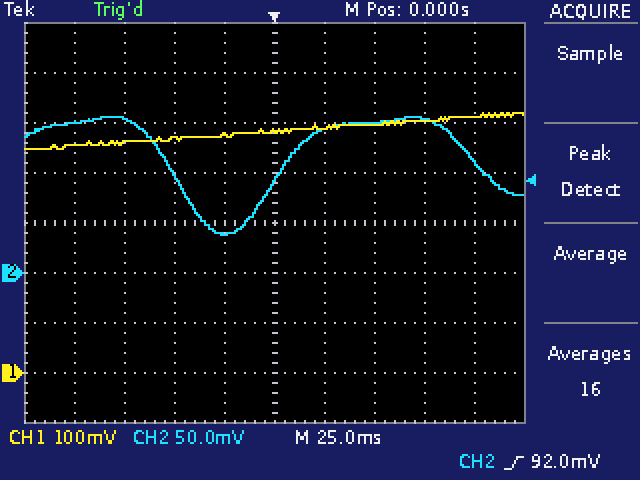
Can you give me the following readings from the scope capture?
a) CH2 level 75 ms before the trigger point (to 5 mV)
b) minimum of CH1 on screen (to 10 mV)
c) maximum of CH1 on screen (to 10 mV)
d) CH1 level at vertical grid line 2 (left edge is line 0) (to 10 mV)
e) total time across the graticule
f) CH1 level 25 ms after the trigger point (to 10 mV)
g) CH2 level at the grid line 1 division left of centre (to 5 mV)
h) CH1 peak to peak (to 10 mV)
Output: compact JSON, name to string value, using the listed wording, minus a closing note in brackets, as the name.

{"CH2 level 75 ms before the trigger point": "155 mV", "minimum of CH1 on screen": "450 mV", "maximum of CH1 on screen": "520 mV", "CH1 level at vertical grid line 2 (left edge is line 0)": "460 mV", "total time across the graticule": "250 ms", "CH1 level 25 ms after the trigger point": "490 mV", "CH2 level at the grid line 1 division left of centre": "40 mV", "CH1 peak to peak": "70 mV"}
